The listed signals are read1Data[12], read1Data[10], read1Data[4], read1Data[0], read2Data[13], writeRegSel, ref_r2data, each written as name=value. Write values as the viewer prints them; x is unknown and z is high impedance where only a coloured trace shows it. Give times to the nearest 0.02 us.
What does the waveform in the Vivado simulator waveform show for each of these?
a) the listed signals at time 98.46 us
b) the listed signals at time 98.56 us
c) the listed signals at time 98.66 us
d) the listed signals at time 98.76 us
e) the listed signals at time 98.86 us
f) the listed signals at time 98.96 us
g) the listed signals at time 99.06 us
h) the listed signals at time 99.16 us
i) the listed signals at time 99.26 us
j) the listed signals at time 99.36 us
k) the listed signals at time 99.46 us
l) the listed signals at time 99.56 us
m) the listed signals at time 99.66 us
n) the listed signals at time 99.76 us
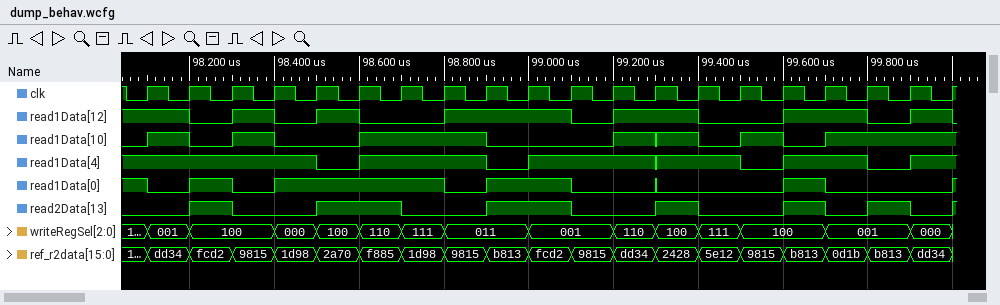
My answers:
read1Data[12]=0, read1Data[10]=0, read1Data[4]=1, read1Data[0]=1, read2Data[13]=0, writeRegSel=000, ref_r2data=1d98
read1Data[12]=1, read1Data[10]=0, read1Data[4]=0, read1Data[0]=1, read2Data[13]=1, writeRegSel=100, ref_r2data=2a70
read1Data[12]=0, read1Data[10]=1, read1Data[4]=1, read1Data[0]=1, read2Data[13]=1, writeRegSel=110, ref_r2data=f885
read1Data[12]=0, read1Data[10]=1, read1Data[4]=1, read1Data[0]=1, read2Data[13]=0, writeRegSel=111, ref_r2data=1d98
read1Data[12]=1, read1Data[10]=1, read1Data[4]=1, read1Data[0]=0, read2Data[13]=0, writeRegSel=011, ref_r2data=9815
read1Data[12]=1, read1Data[10]=0, read1Data[4]=0, read1Data[0]=1, read2Data[13]=1, writeRegSel=011, ref_r2data=b813
read1Data[12]=1, read1Data[10]=0, read1Data[4]=1, read1Data[0]=1, read2Data[13]=1, writeRegSel=001, ref_r2data=fcd2
read1Data[12]=0, read1Data[10]=0, read1Data[4]=1, read1Data[0]=0, read2Data[13]=0, writeRegSel=001, ref_r2data=9815
read1Data[12]=1, read1Data[10]=1, read1Data[4]=1, read1Data[0]=0, read2Data[13]=0, writeRegSel=110, ref_r2data=dd34
read1Data[12]=1, read1Data[10]=1, read1Data[4]=1, read1Data[0]=0, read2Data[13]=1, writeRegSel=100, ref_r2data=2428
read1Data[12]=0, read1Data[10]=0, read1Data[4]=1, read1Data[0]=0, read2Data[13]=0, writeRegSel=111, ref_r2data=5e12
read1Data[12]=0, read1Data[10]=1, read1Data[4]=0, read1Data[0]=0, read2Data[13]=0, writeRegSel=100, ref_r2data=9815
read1Data[12]=1, read1Data[10]=0, read1Data[4]=1, read1Data[0]=1, read2Data[13]=1, writeRegSel=100, ref_r2data=b813
read1Data[12]=1, read1Data[10]=1, read1Data[4]=1, read1Data[0]=0, read2Data[13]=0, writeRegSel=001, ref_r2data=0d1b
